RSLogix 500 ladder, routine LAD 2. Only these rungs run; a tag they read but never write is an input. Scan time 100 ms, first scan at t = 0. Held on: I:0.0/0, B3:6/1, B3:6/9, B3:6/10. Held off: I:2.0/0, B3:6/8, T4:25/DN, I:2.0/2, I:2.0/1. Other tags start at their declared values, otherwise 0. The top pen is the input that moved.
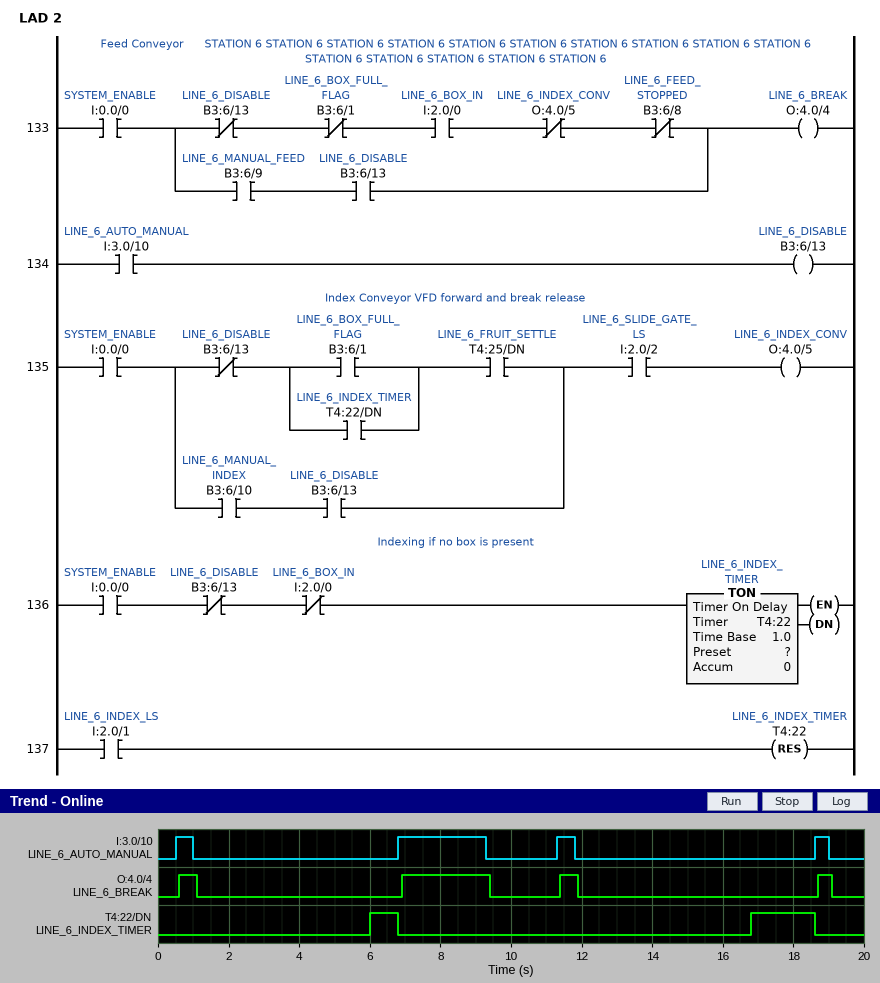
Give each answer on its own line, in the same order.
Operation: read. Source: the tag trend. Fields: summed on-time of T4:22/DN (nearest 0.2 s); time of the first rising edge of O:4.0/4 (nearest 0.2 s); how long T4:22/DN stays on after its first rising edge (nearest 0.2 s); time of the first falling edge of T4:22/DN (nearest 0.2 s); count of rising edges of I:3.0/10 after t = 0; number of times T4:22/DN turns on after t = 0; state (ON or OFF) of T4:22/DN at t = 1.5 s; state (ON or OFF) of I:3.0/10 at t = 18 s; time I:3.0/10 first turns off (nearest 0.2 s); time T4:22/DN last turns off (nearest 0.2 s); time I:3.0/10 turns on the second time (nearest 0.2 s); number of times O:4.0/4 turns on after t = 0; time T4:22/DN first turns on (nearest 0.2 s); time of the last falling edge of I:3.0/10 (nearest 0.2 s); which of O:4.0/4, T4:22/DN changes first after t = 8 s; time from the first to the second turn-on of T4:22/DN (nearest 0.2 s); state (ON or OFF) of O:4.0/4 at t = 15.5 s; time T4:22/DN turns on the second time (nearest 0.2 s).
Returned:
2.6 s
0.6 s
0.8 s
6.8 s
4
2
OFF
OFF
1.0 s
18.6 s
6.8 s
4
6.0 s
19.0 s
O:4.0/4
10.8 s
OFF
16.8 s
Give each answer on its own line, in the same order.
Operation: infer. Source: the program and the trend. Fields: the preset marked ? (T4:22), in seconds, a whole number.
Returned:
5 s
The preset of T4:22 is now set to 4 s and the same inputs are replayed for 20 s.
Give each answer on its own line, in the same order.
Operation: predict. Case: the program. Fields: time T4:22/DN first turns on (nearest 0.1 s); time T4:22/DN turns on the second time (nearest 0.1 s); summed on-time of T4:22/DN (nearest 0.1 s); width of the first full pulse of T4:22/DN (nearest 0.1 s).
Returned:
5.0 s
15.8 s
4.6 s
1.8 s
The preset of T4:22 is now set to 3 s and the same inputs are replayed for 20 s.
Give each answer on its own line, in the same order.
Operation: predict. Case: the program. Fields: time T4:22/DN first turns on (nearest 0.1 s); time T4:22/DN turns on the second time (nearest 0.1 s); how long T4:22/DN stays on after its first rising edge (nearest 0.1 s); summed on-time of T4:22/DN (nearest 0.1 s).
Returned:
4.0 s
14.8 s
2.8 s
6.6 s
